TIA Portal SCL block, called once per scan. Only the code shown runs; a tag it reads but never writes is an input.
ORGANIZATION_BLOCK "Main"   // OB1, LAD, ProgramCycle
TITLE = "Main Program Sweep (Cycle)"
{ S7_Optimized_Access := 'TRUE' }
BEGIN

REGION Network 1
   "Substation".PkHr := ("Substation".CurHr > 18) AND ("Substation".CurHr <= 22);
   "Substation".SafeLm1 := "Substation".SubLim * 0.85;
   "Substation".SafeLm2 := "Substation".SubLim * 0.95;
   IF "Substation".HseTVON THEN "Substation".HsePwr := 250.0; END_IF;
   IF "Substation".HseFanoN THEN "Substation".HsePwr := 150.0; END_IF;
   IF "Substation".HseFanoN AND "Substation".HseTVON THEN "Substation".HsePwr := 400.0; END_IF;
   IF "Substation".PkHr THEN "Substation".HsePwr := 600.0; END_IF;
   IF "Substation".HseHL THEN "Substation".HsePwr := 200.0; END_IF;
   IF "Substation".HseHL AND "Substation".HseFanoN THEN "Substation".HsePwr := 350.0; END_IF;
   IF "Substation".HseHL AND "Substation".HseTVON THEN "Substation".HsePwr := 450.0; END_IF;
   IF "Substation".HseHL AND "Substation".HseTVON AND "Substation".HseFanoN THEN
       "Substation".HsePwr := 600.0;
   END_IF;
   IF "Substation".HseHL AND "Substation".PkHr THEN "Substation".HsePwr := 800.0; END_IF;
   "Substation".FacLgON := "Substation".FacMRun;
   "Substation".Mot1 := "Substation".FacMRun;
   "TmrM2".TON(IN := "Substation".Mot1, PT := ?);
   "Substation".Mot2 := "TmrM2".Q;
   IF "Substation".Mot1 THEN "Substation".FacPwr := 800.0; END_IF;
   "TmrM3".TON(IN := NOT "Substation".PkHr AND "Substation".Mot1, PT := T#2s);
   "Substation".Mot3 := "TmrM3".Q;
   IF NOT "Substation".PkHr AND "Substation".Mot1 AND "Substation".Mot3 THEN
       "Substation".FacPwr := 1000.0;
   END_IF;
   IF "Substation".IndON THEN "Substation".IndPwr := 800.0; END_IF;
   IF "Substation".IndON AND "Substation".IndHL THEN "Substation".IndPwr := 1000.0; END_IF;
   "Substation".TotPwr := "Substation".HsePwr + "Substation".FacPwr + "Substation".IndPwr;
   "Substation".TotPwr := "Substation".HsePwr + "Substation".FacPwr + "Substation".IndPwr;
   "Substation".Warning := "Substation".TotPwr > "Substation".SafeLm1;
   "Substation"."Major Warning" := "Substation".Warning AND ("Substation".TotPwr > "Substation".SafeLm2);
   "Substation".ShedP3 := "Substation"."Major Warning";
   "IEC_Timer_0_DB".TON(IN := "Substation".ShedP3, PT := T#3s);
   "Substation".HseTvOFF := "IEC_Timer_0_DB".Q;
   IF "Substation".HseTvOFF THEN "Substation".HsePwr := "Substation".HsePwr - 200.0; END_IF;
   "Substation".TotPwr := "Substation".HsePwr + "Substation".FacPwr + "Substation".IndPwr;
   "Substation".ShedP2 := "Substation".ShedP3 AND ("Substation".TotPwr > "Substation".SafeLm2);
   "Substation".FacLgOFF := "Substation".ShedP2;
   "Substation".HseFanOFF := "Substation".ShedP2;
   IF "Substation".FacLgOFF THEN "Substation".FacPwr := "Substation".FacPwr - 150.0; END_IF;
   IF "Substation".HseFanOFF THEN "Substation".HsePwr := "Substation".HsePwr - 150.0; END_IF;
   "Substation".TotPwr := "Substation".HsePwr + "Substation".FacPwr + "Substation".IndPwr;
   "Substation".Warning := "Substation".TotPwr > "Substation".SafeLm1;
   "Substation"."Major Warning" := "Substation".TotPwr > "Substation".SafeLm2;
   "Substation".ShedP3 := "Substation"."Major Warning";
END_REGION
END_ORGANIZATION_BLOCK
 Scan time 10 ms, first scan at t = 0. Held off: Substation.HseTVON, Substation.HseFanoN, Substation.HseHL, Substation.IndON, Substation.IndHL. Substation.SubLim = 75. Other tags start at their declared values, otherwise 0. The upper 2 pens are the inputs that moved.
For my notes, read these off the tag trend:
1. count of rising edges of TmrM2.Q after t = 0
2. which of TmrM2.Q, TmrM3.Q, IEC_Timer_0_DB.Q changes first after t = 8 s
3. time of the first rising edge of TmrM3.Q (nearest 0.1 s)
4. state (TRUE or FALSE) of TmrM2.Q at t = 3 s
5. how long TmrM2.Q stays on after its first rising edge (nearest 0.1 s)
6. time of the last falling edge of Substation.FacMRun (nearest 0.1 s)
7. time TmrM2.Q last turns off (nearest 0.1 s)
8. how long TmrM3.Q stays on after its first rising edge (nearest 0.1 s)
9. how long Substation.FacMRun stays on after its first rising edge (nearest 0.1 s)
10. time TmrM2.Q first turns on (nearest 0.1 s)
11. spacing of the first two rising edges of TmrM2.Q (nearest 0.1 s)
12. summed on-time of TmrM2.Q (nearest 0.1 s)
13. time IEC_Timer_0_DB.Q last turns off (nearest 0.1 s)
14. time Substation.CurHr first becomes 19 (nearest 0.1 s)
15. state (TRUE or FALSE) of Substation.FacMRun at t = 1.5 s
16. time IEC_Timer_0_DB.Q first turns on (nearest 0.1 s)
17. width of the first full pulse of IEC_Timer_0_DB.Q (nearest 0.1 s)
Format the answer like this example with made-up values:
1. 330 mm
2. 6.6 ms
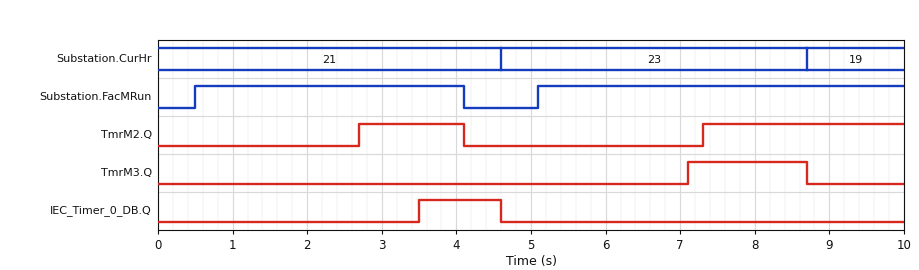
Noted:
1. 2
2. TmrM3.Q
3. 7.1 s
4. TRUE
5. 1.4 s
6. 4.1 s
7. 4.1 s
8. 1.6 s
9. 3.6 s
10. 2.7 s
11. 4.6 s
12. 4.1 s
13. 4.6 s
14. 8.7 s
15. TRUE
16. 3.5 s
17. 1.1 s
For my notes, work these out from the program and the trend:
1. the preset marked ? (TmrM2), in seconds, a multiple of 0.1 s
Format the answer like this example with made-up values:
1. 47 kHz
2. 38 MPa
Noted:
1. 2.2 s
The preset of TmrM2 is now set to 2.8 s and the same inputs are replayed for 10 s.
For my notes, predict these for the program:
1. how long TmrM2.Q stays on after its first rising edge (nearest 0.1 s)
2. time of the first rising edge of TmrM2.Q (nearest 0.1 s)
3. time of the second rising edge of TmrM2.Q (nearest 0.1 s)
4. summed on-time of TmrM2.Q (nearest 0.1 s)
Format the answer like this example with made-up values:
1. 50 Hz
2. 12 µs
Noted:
1. 0.8 s
2. 3.3 s
3. 7.9 s
4. 2.9 s
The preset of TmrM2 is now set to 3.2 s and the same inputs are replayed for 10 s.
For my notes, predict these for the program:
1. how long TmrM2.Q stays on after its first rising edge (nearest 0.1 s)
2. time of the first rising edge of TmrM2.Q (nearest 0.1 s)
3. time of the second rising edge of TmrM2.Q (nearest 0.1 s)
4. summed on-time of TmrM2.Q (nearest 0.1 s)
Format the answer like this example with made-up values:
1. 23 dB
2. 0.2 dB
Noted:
1. 0.4 s
2. 3.7 s
3. 8.3 s
4. 2.1 s
